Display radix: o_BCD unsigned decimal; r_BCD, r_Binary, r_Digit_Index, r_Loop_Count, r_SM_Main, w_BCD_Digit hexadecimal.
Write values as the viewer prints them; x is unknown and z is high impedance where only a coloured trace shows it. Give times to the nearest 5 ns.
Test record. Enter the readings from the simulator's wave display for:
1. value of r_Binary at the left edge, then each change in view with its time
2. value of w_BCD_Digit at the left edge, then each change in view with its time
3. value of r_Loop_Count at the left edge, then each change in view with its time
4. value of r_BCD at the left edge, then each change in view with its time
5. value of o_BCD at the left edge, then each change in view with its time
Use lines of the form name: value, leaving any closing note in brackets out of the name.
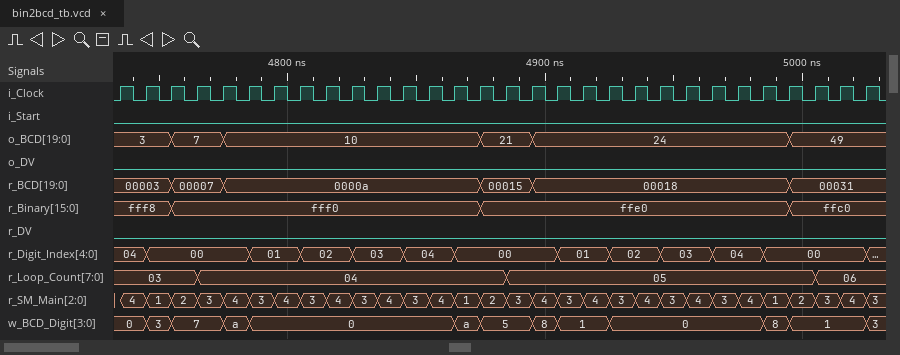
value of r_Binary at the left edge, then each change in view with its time: fff8, fff0 at 4755 ns, ffe0 at 4875 ns, ffc0 at 4995 ns
value of w_BCD_Digit at the left edge, then each change in view with its time: 0, 3 at 4745 ns, 7 at 4755 ns, a at 4775 ns, 0 at 4785 ns, a at 4865 ns, 5 at 4875 ns, 8 at 4895 ns, 1 at 4905 ns, 0 at 4925 ns, 8 at 4985 ns, 1 at 4995 ns, 3 at 5025 ns
value of r_Loop_Count at the left edge, then each change in view with its time: 03, 04 at 4765 ns, 05 at 4885 ns, 06 at 5005 ns
value of r_BCD at the left edge, then each change in view with its time: 00003, 00007 at 4755 ns, 0000a at 4775 ns, 00015 at 4875 ns, 00018 at 4895 ns, 00031 at 4995 ns
value of o_BCD at the left edge, then each change in view with its time: 3, 7 at 4755 ns, 10 at 4775 ns, 21 at 4875 ns, 24 at 4895 ns, 49 at 4995 ns
